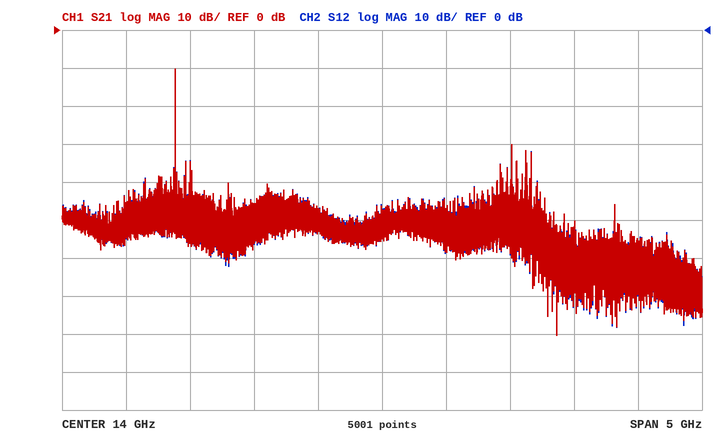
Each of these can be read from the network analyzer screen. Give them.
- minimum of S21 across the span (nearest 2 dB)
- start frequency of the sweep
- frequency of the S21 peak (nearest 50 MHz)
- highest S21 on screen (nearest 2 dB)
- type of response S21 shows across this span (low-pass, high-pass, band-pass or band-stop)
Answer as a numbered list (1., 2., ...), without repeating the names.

1. -80 dB
2. 11.5 GHz
3. 12.40 GHz
4. -10 dB
5. band-pass
